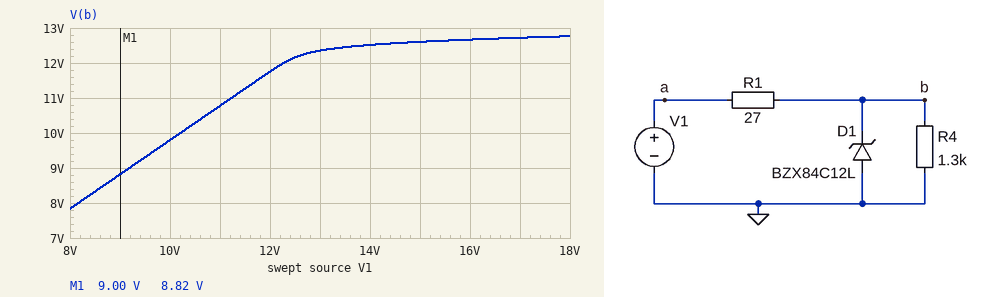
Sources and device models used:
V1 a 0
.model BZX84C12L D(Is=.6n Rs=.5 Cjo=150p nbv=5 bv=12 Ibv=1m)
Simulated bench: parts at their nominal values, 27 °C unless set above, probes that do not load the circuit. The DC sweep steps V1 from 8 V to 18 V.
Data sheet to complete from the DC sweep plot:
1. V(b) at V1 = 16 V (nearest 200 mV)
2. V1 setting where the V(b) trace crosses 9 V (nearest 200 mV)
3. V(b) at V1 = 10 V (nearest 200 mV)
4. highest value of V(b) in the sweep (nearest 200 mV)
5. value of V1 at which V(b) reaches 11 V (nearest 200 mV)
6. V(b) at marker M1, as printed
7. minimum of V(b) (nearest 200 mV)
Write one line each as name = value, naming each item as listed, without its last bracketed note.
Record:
V(b) at V1 = 16 V = 12.6 V
V1 setting where the V(b) trace crosses 9 V = 9.2 V
V(b) at V1 = 10 V = 9.8 V
highest value of V(b) in the sweep = 12.8 V
value of V1 at which V(b) reaches 11 V = 11.2 V
V(b) at marker M1, as printed = 8.82 V
minimum of V(b) = 7.8 V
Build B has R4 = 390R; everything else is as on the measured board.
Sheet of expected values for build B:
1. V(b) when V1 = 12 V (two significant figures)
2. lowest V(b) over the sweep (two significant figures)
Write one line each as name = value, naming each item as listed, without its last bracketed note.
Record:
V(b) when V1 = 12 V = 11 V
lowest V(b) over the sweep = 7.5 V
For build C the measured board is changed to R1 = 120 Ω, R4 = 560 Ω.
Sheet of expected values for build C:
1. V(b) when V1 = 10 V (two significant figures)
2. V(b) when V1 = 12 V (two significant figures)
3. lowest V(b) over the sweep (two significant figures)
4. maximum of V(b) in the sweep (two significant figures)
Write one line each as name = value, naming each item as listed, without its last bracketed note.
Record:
V(b) when V1 = 10 V = 8.2 V
V(b) when V1 = 12 V = 9.9 V
lowest V(b) over the sweep = 6.6 V
maximum of V(b) in the sweep = 12 V
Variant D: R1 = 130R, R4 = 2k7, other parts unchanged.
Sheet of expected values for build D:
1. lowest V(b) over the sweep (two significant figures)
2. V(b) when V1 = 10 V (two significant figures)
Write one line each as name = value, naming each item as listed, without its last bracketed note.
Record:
lowest V(b) over the sweep = 7.6 V
V(b) when V1 = 10 V = 9.5 V
